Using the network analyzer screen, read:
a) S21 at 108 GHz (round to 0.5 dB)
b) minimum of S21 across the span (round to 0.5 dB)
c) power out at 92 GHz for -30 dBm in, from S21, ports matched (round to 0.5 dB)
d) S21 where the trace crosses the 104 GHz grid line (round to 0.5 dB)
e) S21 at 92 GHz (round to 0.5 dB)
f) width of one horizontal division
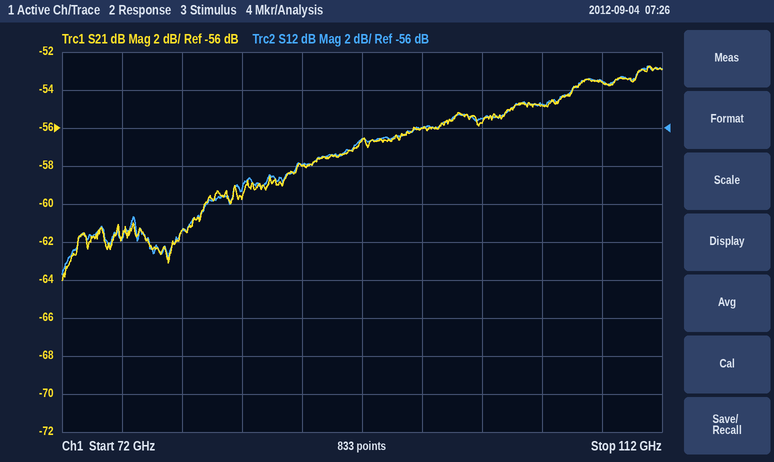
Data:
-53.5 dB
-64.0 dB
-86.5 dBm
-55.0 dB
-56.5 dB
4 GHz
